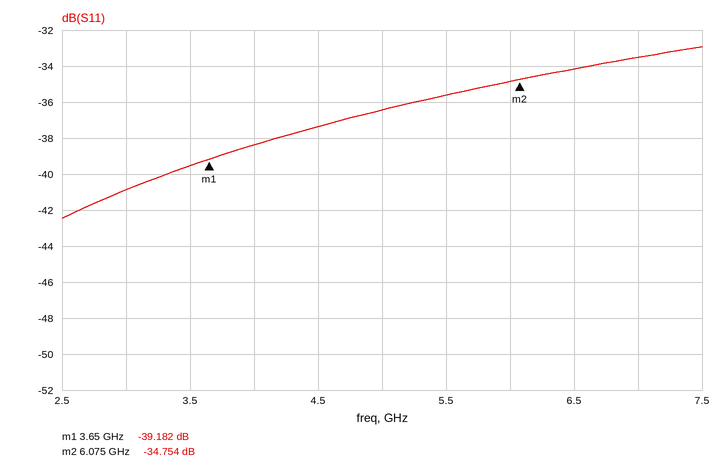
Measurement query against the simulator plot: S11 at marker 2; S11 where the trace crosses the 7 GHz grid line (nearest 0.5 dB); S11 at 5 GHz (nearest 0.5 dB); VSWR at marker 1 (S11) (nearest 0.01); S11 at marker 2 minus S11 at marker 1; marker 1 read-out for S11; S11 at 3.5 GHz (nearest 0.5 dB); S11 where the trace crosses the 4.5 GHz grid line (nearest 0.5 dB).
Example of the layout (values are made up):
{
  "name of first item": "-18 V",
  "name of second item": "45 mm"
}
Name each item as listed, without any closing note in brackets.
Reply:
{
  "S11 at marker 2": "-34.754 dB",
  "S11 where the trace crosses the 7 GHz grid line": "-33.5 dB",
  "S11 at 5 GHz": "-36.5 dB",
  "VSWR at marker 1 (S11)": "1.02",
  "S11 at marker 2 minus S11 at marker 1": "4.428 dB",
  "marker 1 read-out for S11": "-39.182 dB",
  "S11 at 3.5 GHz": "-39.5 dB",
  "S11 where the trace crosses the 4.5 GHz grid line": "-37.5 dB"
}
